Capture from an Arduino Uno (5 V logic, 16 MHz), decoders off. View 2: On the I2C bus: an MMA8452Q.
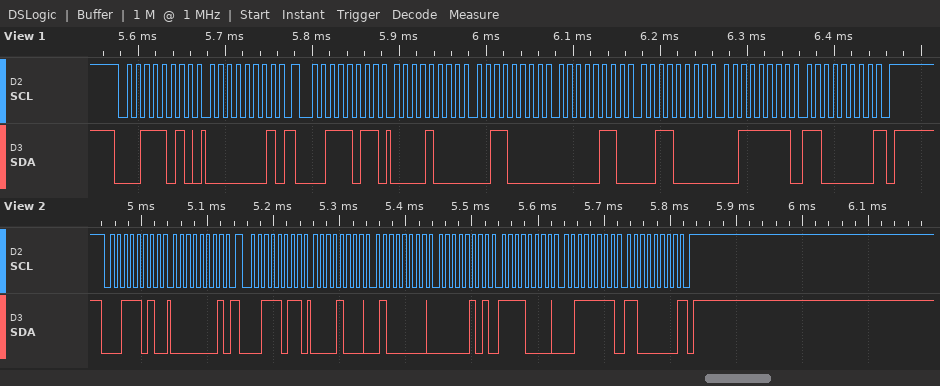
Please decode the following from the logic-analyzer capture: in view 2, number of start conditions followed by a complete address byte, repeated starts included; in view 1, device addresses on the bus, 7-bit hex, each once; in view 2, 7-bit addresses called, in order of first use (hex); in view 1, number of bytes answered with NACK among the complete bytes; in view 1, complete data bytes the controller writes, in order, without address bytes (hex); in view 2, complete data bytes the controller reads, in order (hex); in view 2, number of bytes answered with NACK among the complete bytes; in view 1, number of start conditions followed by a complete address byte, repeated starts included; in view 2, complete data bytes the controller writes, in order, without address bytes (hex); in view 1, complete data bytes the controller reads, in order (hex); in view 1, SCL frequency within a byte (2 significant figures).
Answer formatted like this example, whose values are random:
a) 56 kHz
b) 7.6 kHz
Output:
a) 2
b) 0x1D
c) 0x1D
d) 1
e) 01
f) 08 40 05 F0 3F C0
g) 1
h) 2
i) 01
j) 08 30 06 30 3F C0
k) 100 kHz
